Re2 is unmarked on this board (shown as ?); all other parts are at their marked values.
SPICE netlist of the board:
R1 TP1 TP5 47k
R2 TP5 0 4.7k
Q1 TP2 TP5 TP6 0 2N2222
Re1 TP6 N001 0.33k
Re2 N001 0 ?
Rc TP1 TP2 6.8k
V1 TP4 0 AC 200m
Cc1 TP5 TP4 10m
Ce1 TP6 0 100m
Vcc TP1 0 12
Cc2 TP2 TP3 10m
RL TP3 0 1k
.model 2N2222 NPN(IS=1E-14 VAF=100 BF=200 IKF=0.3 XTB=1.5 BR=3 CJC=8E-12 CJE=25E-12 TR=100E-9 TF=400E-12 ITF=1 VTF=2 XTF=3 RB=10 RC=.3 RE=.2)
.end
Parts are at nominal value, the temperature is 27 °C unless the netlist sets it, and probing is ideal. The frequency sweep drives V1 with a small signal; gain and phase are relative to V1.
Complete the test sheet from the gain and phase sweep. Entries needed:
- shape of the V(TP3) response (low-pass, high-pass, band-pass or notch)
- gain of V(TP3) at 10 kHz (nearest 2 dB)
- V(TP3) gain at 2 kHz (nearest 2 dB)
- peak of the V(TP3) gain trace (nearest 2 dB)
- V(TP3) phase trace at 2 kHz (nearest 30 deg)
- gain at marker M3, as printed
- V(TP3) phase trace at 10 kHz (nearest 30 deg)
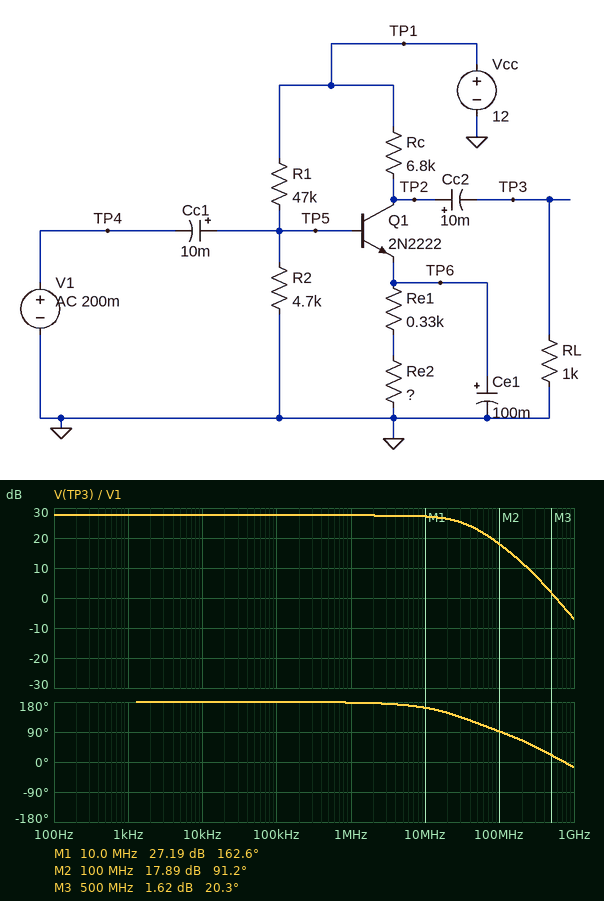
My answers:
low-pass
28 dB
28 dB
28 dB
180 deg
1.62 dB
180 deg
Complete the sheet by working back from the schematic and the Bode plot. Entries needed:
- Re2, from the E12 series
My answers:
270 Ω
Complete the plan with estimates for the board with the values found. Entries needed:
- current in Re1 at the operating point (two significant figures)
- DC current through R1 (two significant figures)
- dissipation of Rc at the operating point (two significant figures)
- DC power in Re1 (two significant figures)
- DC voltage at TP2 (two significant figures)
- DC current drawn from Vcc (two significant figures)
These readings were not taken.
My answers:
720 µA
230 µA
3.5 mW
170 µW
7.1 V
950 µA
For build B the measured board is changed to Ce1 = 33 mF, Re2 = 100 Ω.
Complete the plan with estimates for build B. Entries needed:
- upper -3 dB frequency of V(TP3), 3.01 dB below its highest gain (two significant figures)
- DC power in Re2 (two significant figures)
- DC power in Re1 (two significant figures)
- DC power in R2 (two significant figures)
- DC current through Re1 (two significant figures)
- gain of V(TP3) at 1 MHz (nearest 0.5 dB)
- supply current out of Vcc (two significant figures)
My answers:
30 MHz
94 µW
310 µW
240 µW
970 µA
30.0 dB
1.2 mA
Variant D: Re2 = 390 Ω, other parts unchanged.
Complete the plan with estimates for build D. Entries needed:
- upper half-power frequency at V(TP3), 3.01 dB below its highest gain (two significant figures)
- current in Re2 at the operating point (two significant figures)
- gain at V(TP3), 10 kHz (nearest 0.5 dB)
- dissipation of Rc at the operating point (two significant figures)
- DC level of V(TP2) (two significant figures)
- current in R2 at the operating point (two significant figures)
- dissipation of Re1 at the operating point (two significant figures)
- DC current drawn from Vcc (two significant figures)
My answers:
38 MHz
610 µA
26.0 dB
2.5 mW
7.9 V
230 µA
120 µW
840 µA
